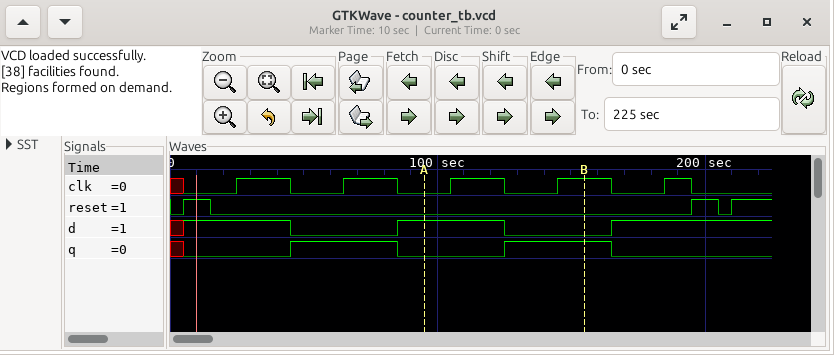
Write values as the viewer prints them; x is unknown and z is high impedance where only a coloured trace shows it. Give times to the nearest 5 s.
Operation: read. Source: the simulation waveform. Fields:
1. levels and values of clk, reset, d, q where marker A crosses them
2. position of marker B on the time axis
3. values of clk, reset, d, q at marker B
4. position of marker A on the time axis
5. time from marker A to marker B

clk=0, reset=0, d=1, q=0
155 s
clk=1, reset=0, d=0, q=1
95 s
60 s
